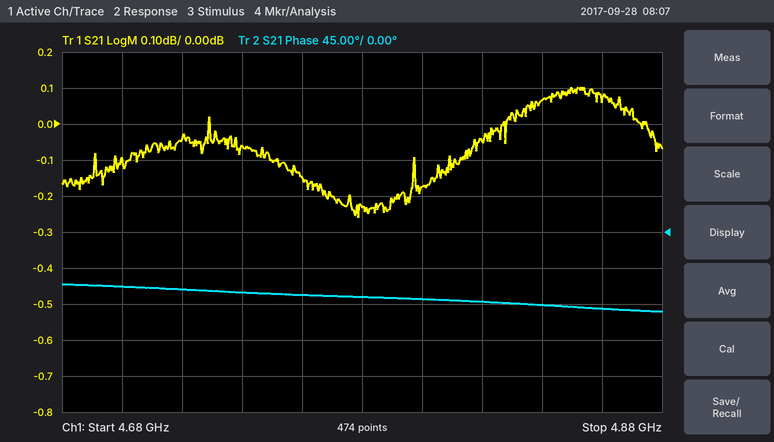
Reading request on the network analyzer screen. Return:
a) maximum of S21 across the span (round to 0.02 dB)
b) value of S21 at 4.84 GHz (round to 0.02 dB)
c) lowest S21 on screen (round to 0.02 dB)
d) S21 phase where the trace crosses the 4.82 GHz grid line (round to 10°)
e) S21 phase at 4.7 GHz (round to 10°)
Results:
0.10 dB
0.06 dB
-0.26 dB
-90°
-70°
